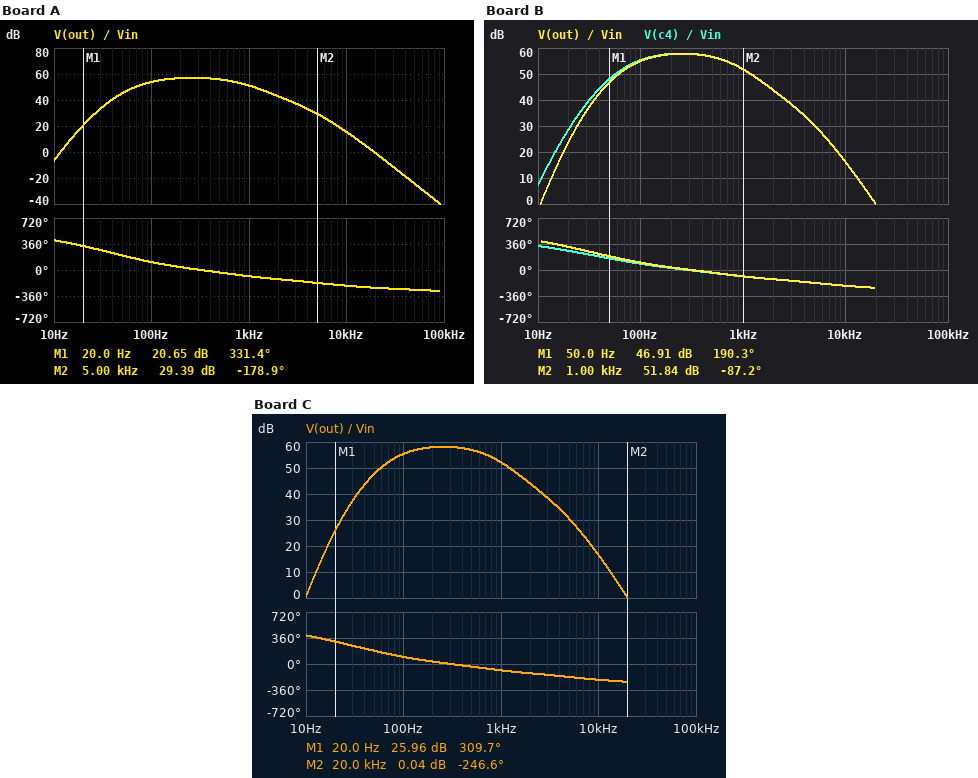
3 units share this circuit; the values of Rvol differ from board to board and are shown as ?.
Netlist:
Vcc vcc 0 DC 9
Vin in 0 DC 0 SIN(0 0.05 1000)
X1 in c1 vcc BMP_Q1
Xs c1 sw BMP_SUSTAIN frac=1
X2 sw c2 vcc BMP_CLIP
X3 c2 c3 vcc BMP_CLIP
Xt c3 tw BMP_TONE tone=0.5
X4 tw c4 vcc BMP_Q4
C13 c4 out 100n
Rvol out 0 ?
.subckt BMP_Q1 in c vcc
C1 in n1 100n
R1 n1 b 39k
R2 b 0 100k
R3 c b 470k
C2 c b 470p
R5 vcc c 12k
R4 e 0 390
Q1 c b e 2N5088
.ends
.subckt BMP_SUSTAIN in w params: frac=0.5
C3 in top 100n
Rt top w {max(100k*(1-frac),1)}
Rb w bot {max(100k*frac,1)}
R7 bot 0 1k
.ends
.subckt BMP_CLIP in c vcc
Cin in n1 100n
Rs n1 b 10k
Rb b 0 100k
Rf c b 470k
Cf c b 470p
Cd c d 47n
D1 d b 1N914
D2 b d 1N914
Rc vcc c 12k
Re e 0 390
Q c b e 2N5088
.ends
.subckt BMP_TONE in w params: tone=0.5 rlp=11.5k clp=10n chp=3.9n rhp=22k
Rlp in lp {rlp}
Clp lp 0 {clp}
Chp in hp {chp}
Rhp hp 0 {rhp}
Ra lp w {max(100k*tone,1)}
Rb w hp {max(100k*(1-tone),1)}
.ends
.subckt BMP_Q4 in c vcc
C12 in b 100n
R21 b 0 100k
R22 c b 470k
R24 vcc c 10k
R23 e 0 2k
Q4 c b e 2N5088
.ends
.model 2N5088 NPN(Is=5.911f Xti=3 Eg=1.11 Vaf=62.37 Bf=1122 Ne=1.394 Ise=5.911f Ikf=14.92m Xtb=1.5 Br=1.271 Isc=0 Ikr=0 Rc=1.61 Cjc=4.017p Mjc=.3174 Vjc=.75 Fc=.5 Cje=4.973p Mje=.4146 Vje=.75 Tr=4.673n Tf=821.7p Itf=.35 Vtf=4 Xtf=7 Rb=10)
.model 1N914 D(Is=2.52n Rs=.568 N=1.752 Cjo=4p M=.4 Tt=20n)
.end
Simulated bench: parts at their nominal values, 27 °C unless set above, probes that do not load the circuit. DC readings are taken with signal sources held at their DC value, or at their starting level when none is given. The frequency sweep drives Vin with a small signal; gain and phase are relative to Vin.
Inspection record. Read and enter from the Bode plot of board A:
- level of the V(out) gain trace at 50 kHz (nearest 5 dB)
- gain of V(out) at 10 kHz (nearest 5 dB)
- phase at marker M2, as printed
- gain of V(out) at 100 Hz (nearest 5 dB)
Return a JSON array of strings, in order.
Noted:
["-25 dB", "15 dB", "-178.9 deg", "55 dB"]
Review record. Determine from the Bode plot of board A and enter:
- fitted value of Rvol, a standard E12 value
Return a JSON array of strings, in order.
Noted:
["33 kΩ"]
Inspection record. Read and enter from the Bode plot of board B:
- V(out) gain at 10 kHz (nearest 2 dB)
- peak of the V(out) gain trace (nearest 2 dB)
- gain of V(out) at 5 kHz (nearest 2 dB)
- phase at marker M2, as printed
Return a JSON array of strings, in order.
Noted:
["16 dB", "58 dB", "30 dB", "-87.2 deg"]
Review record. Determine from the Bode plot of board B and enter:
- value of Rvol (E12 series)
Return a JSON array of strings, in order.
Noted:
["56 kΩ"]
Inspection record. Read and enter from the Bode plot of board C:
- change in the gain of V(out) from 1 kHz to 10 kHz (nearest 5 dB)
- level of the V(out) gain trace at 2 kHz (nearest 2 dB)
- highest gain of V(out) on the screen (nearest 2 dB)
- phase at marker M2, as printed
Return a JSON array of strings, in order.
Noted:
["-35 dB", "44 dB", "58 dB", "-246.6 deg"]
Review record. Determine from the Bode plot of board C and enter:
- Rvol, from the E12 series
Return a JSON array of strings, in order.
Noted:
["82 kΩ"]
